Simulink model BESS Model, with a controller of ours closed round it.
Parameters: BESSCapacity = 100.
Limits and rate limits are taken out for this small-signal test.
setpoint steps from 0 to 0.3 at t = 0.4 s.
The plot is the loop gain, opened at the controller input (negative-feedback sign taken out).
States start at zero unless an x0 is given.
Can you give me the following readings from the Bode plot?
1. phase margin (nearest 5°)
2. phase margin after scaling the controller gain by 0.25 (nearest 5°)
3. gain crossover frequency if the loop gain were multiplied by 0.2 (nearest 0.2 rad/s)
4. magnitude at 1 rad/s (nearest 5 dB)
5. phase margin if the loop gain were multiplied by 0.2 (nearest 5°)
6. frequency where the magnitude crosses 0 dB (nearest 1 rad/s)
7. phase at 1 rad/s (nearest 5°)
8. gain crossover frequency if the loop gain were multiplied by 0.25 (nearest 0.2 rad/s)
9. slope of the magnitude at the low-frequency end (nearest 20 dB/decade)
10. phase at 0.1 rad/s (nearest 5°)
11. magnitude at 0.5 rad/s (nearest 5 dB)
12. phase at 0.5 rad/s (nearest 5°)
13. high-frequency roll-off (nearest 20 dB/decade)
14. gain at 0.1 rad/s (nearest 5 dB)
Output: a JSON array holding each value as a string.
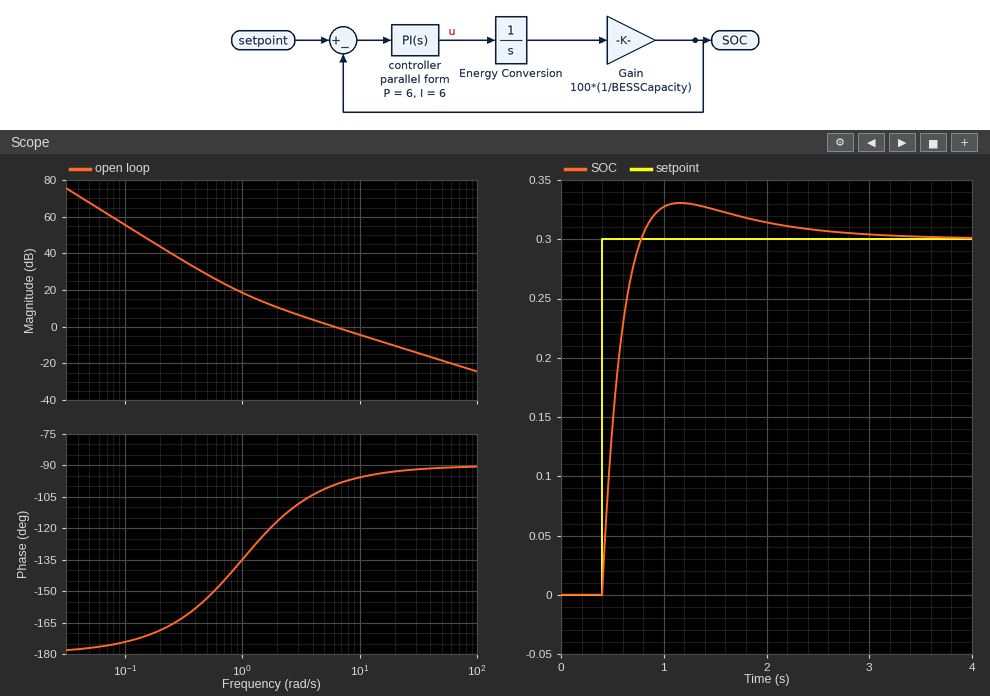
["80°", "60°", "1.4 rad/s", "20 dB", "55°", "6 rad/s", "-135°", "1.8 rad/s", "-40 dB/decade", "-175°", "30 dB", "-155°", "-20 dB/decade", "55 dB"]
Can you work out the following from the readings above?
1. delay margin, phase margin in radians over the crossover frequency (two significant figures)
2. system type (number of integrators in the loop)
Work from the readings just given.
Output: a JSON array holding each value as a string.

["0.23 s", "2"]
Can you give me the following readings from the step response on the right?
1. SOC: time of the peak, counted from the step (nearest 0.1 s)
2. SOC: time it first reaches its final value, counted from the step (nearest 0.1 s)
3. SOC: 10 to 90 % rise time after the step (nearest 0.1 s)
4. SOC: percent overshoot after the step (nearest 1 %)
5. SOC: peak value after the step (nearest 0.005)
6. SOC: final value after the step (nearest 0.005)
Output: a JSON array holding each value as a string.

["0.8 s", "0.4 s", "0.3 s", "10 %", "0.330", "0.300"]
